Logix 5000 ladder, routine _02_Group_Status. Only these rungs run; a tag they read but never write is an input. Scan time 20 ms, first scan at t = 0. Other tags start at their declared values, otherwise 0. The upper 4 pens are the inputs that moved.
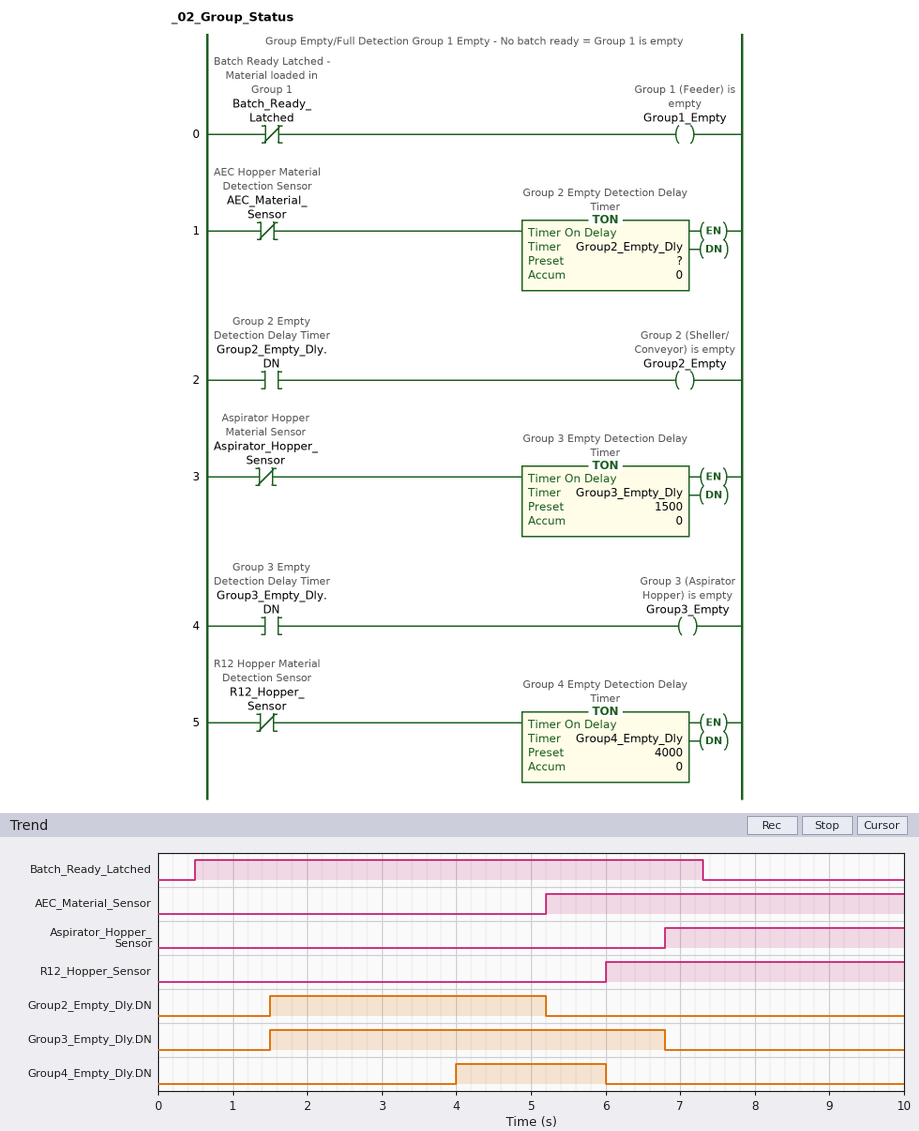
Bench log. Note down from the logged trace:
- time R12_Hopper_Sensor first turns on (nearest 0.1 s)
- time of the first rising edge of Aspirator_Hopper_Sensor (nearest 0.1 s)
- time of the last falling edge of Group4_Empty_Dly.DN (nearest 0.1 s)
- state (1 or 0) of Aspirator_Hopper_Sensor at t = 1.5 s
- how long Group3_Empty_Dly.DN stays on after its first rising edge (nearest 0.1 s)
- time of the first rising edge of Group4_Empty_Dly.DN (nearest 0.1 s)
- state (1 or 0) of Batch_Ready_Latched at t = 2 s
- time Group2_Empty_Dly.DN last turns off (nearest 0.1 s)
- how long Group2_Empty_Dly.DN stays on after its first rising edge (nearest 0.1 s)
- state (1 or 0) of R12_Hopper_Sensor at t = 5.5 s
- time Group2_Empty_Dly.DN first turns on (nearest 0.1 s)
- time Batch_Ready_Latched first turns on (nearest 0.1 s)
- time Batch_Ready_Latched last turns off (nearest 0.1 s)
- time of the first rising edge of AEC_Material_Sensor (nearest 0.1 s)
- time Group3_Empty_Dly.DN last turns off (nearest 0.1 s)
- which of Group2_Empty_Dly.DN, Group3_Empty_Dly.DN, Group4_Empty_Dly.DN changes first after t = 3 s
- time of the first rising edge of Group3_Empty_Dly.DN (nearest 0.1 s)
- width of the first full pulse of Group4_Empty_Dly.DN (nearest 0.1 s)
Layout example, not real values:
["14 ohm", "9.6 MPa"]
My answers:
["6.0 s", "6.8 s", "6.0 s", "0", "5.3 s", "4.0 s", "1", "5.2 s", "3.7 s", "0", "1.5 s", "0.5 s", "7.3 s", "5.2 s", "6.8 s", "Group4_Empty_Dly.DN", "1.5 s", "2.0 s"]
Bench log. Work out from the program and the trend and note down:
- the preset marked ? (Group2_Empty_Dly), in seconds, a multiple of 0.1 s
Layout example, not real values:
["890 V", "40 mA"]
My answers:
["1.5 s"]
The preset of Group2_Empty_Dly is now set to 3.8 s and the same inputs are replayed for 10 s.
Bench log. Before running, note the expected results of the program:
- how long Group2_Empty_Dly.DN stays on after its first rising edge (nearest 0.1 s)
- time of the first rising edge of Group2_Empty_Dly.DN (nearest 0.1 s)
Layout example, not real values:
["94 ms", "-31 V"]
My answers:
["1.4 s", "3.8 s"]
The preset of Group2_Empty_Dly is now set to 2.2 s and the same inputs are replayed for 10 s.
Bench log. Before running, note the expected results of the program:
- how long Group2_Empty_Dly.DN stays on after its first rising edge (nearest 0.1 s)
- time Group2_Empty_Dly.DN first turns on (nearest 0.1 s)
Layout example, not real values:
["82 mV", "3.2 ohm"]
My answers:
["3.0 s", "2.2 s"]
